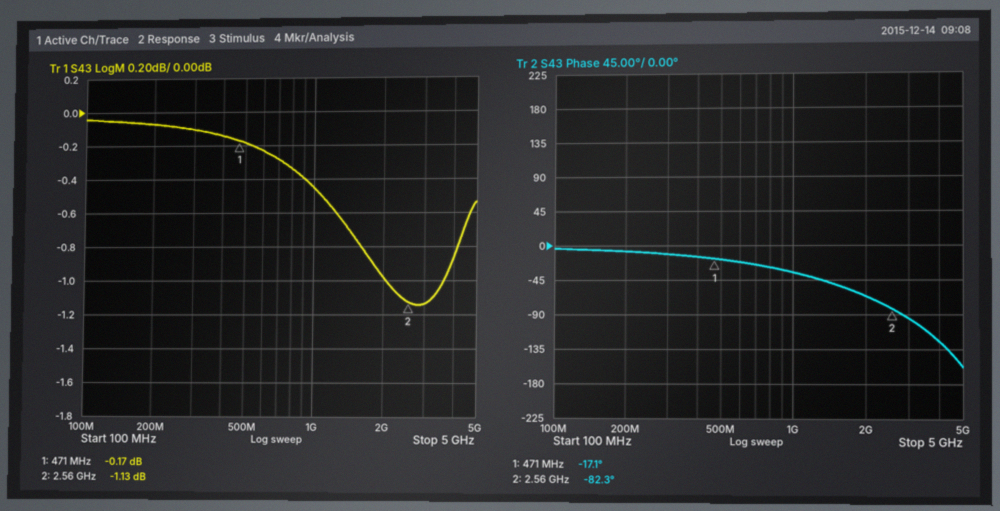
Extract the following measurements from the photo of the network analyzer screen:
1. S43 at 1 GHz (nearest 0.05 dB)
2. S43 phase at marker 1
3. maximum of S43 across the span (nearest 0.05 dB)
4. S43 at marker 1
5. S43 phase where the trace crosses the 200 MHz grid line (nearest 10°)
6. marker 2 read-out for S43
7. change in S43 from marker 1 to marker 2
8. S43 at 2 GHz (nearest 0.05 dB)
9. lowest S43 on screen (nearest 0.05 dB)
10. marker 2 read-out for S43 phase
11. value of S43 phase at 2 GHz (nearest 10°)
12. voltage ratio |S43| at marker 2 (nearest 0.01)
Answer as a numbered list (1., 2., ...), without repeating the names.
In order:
1. -0.45 dB
2. -17.1°
3. -0.05 dB
4. -0.17 dB
5. -10°
6. -1.13 dB
7. -0.96 dB
8. -1.00 dB
9. -1.15 dB
10. -82.3°
11. -70°
12. 0.88
